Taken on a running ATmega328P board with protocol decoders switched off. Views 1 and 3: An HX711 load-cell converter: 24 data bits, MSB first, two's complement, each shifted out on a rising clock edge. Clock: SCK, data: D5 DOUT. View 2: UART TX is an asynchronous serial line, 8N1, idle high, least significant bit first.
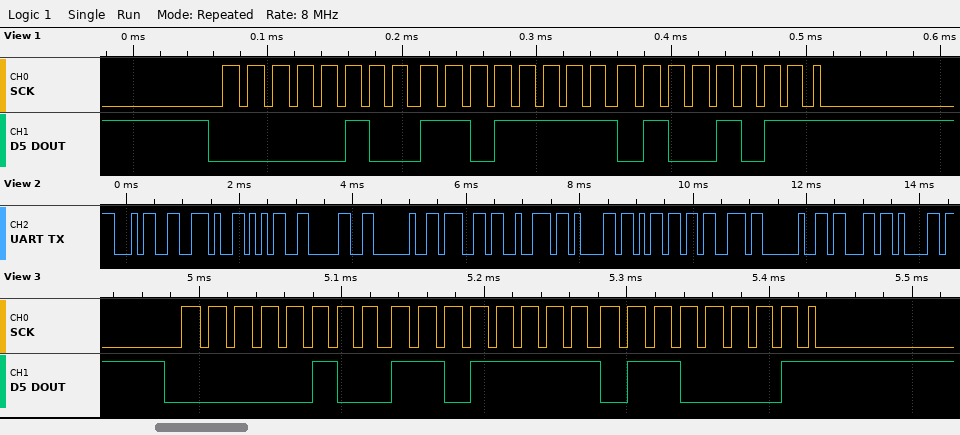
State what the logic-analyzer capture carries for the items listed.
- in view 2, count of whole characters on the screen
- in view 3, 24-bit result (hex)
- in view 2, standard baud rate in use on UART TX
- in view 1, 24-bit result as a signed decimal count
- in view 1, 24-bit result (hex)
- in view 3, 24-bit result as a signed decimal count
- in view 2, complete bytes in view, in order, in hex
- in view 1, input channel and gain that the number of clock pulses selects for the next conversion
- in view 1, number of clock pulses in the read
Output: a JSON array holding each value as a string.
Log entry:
["13", "0x04DF61", "9600 baud", "319307", "0x04DF4B", "319329", "0x34 0x2E 0x35 0x30 0x20 0x67 0x72 0x61 0x6D 0x73 0x20 0x63 0x61", "channel A, gain 128", "25"]
